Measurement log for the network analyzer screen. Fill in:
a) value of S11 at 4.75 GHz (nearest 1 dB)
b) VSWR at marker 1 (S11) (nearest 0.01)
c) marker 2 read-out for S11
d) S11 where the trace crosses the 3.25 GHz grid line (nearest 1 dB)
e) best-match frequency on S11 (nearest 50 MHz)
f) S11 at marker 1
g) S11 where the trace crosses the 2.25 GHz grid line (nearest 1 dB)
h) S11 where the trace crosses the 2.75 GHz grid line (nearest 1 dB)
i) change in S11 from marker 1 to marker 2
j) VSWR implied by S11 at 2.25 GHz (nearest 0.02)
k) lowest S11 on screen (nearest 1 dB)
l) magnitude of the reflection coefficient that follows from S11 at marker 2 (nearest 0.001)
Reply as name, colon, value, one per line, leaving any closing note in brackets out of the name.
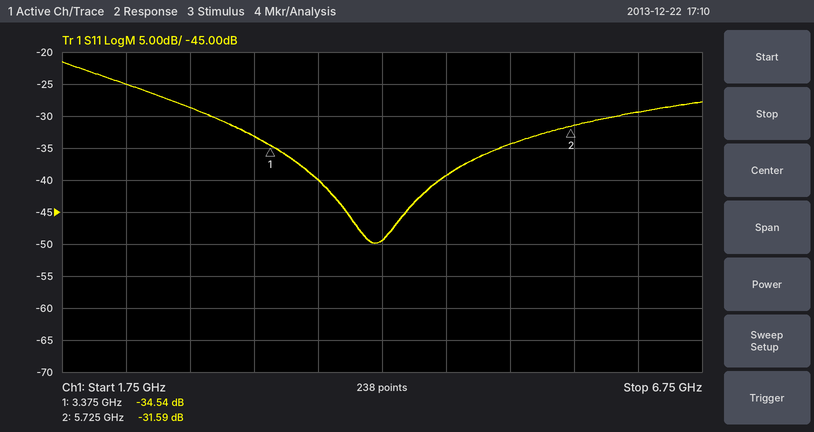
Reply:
value of S11 at 4.75 GHz: -39 dB
VSWR at marker 1 (S11): 1.04
marker 2 read-out for S11: -31.59 dB
S11 where the trace crosses the 3.25 GHz grid line: -33 dB
best-match frequency on S11: 4.20 GHz
S11 at marker 1: -34.54 dB
S11 where the trace crosses the 2.25 GHz grid line: -25 dB
S11 where the trace crosses the 2.75 GHz grid line: -29 dB
change in S11 from marker 1 to marker 2: 2.95 dB
VSWR implied by S11 at 2.25 GHz: 1.12
lowest S11 on screen: -50 dB
magnitude of the reflection coefficient that follows from S11 at marker 2: 0.026
